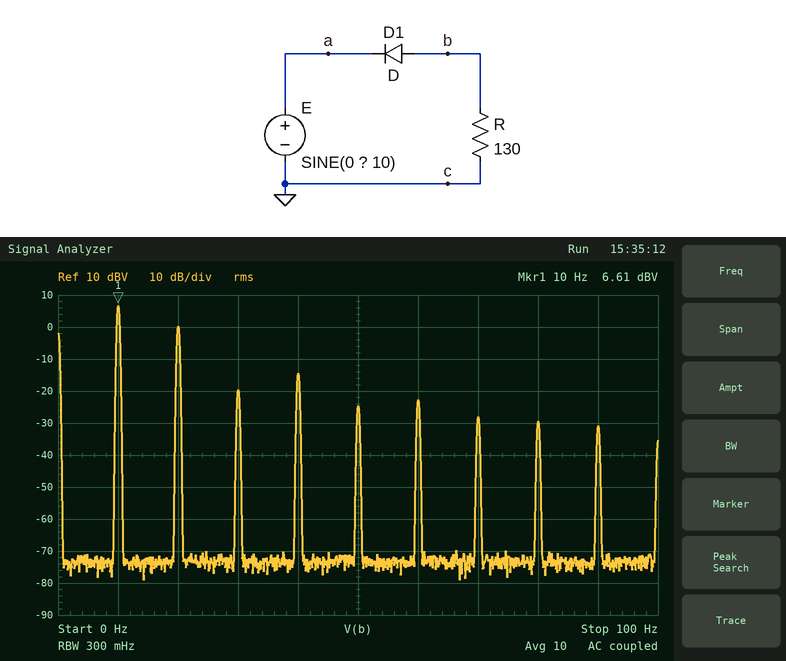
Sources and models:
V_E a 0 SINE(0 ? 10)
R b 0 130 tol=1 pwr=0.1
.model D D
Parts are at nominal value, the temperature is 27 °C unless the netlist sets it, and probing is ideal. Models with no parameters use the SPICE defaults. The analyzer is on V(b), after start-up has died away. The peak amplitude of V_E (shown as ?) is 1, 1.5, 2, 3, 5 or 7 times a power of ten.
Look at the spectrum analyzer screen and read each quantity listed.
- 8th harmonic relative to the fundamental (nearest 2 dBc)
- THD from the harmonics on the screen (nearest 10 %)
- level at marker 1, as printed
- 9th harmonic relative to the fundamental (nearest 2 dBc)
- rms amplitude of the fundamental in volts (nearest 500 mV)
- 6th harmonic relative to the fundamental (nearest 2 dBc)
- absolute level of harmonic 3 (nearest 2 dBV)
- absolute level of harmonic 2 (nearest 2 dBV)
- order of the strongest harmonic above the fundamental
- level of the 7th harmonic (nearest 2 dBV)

-36 dBc
50 %
6.61 dBV
-38 dBc
2.0 V
-30 dBc
-20 dBV
0 dBV
2
-28 dBV
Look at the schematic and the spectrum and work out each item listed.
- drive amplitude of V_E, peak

7 V
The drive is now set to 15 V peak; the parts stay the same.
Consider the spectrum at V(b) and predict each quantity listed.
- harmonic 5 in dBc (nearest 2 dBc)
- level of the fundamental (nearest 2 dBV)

-38 dBc
14 dBV
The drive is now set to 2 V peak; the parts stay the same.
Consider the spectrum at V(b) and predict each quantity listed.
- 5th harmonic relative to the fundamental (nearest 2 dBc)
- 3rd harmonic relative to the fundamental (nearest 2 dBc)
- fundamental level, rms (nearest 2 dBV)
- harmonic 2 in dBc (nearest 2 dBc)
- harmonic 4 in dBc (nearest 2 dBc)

-22 dBc
-14 dBc
-8 dBV
-4 dBc
-28 dBc
